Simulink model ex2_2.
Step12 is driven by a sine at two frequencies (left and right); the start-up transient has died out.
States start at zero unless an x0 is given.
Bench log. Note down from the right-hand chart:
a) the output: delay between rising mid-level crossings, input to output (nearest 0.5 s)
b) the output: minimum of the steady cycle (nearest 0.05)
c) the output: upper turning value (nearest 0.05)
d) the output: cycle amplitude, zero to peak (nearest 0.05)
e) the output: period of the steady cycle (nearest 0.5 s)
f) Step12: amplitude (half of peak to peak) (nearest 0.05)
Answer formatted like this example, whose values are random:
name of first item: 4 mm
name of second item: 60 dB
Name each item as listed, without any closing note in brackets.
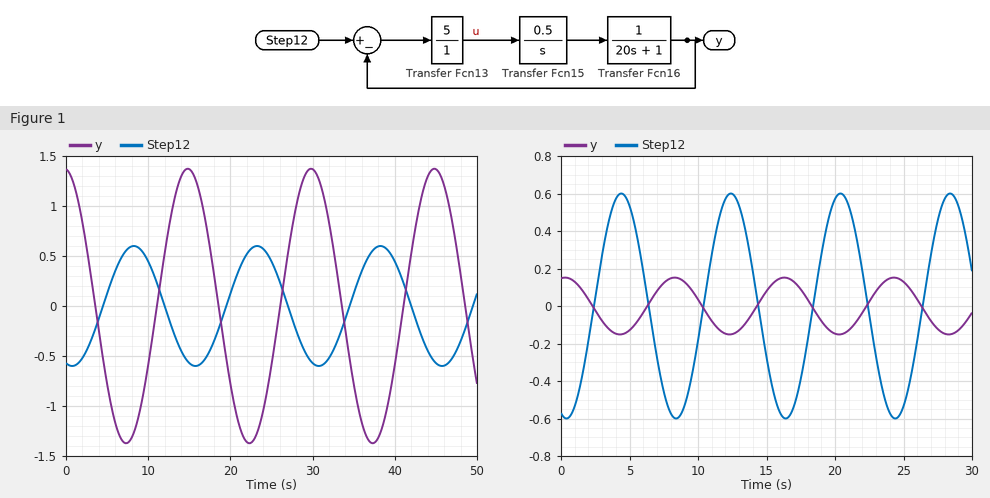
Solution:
the output: delay between rising mid-level crossings, input to output: 4.0 s
the output: minimum of the steady cycle: -0.15
the output: upper turning value: 0.15
the output: cycle amplitude, zero to peak: 0.15
the output: period of the steady cycle: 8.0 s
Step12: amplitude (half of peak to peak): 0.60
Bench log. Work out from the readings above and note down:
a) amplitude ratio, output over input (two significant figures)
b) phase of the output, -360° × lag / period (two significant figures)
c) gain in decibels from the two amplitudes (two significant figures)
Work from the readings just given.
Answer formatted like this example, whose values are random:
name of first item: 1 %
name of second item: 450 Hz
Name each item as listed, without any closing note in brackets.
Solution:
amplitude ratio, output over input: 0.25
phase of the output, -360° × lag / period: -180°
gain in decibels from the two amplitudes: -12 dB
